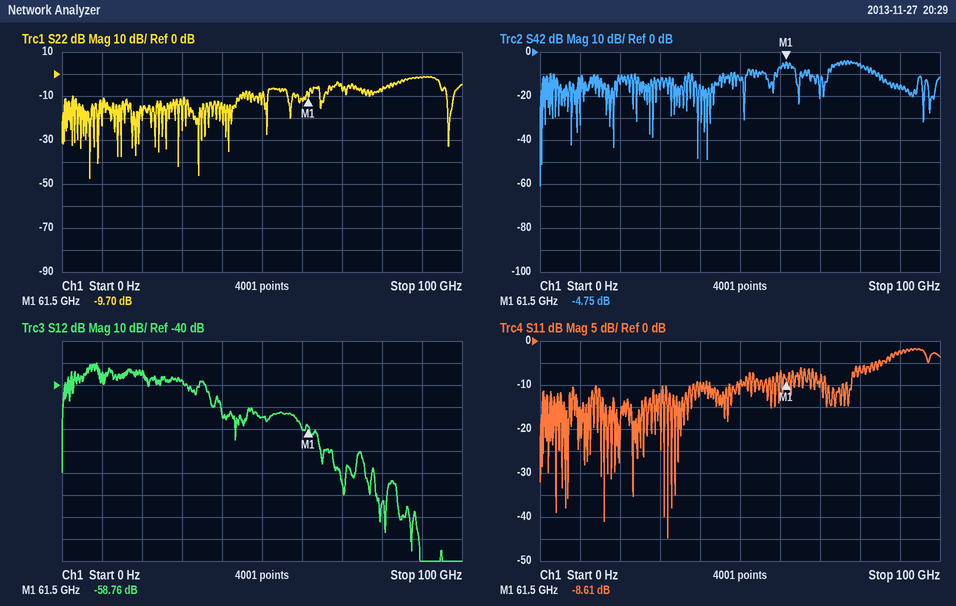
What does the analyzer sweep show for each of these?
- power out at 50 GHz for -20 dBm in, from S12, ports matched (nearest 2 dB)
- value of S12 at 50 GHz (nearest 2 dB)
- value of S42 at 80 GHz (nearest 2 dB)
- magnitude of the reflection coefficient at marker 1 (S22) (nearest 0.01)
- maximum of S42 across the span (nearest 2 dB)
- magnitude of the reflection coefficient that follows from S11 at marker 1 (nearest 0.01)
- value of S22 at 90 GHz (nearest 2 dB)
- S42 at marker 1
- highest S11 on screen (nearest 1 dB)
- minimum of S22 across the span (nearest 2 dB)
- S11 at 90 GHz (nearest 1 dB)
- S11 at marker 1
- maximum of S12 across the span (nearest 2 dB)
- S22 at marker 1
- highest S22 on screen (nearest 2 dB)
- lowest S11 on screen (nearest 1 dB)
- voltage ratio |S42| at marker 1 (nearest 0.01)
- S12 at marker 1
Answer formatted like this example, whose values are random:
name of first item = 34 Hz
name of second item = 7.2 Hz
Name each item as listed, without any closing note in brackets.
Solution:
power out at 50 GHz for -20 dBm in, from S12, ports matched = -74 dBm
value of S12 at 50 GHz = -54 dB
value of S42 at 80 GHz = -6 dB
magnitude of the reflection coefficient at marker 1 (S22) = 0.33
maximum of S42 across the span = -4 dB
magnitude of the reflection coefficient that follows from S11 at marker 1 = 0.37
value of S22 at 90 GHz = -2 dB
S42 at marker 1 = -4.75 dB
highest S11 on screen = -2 dB
minimum of S22 across the span = -48 dB
S11 at 90 GHz = -2 dB
S11 at marker 1 = -8.61 dB
maximum of S12 across the span = -30 dB
S22 at marker 1 = -9.70 dB
highest S22 on screen = -2 dB
lowest S11 on screen = -45 dB
voltage ratio |S42| at marker 1 = 0.58
S12 at marker 1 = -58.76 dB
